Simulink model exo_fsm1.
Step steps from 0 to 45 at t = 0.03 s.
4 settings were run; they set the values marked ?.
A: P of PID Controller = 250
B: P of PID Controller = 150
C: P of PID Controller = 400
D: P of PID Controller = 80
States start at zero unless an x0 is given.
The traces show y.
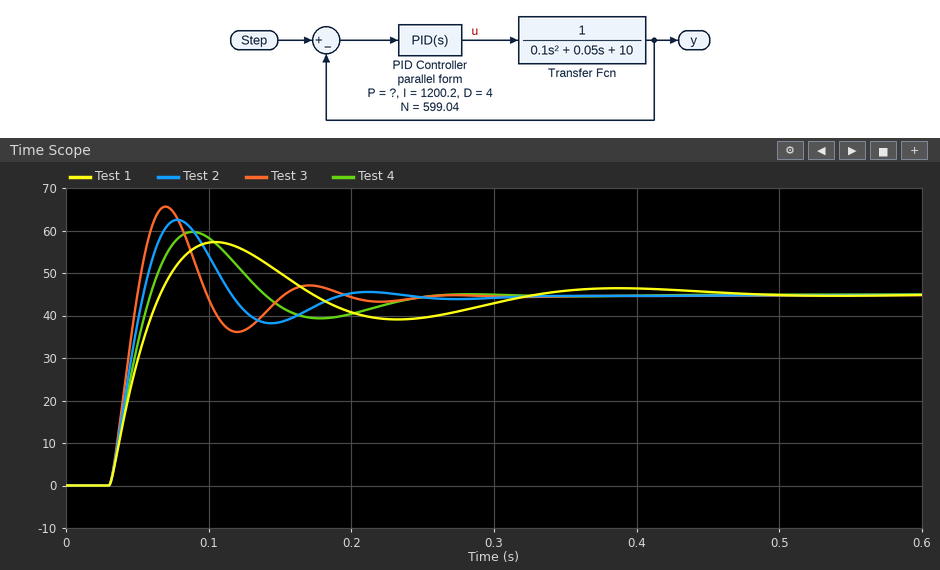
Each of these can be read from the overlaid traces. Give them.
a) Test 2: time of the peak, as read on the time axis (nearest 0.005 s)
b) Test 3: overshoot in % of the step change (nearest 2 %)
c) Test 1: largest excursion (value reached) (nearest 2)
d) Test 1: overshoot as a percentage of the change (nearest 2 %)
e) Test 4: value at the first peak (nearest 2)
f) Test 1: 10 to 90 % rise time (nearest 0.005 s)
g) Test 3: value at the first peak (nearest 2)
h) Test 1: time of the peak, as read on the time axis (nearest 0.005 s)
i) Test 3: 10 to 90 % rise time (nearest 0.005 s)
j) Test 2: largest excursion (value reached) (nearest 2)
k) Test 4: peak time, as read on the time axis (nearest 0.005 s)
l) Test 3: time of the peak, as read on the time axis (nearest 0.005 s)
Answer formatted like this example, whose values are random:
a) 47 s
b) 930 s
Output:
a) 0.080 s
b) 46 %
c) 58
d) 28 %
e) 60
f) 0.025 s
g) 66
h) 0.105 s
i) 0.015 s
j) 62
k) 0.090 s
l) 0.070 s
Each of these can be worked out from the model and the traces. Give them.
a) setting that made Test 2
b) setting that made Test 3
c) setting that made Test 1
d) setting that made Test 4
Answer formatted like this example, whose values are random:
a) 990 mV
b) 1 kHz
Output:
a) A
b) C
c) D
d) B
